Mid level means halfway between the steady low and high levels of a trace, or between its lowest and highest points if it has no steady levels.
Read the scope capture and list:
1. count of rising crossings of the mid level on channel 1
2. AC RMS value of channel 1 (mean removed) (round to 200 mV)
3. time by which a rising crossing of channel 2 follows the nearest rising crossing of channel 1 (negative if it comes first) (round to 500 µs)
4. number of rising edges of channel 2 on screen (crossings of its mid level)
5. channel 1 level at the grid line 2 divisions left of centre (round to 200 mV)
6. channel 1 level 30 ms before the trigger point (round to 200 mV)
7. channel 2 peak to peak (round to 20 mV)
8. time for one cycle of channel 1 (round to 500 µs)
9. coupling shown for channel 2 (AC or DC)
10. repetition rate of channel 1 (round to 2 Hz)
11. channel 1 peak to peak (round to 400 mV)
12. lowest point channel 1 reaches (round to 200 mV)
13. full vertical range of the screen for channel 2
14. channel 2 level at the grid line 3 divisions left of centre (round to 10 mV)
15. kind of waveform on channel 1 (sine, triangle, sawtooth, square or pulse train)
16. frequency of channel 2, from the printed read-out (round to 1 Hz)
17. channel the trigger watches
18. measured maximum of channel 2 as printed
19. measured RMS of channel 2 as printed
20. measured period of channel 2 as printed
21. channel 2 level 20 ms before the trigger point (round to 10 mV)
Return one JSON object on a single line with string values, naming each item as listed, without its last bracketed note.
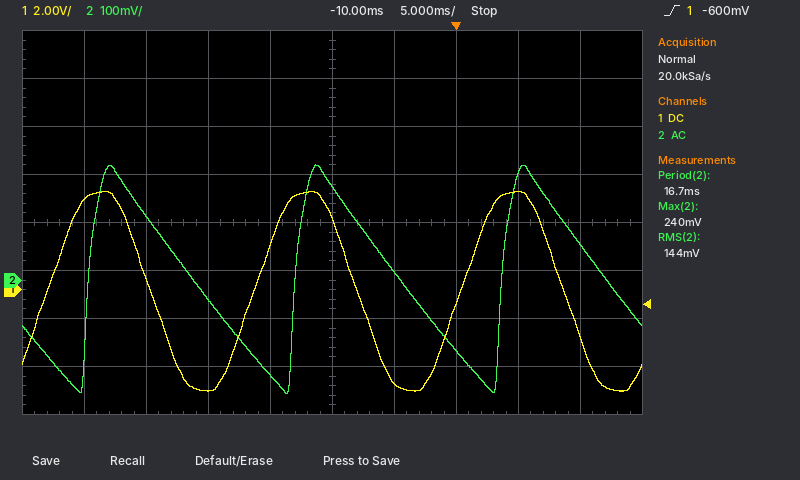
{"count of rising crossings of the mid level on channel 1": "3", "AC RMS value of channel 1 (mean removed)": "3.0 V", "time by which a rising crossing of channel 2 follows the nearest rising crossing of channel 1 (negative if it comes first)": "+3.5 ms", "number of rising edges of channel 2 on screen": "3", "channel 1 level at the grid line 2 divisions left of centre": "-4.2 V", "channel 1 level 30 ms before the trigger point": "3.8 V", "channel 2 peak to peak": "480 mV", "time for one cycle of channel 1": "16.5 ms", "coupling shown for channel 2": "AC", "repetition rate of channel 1": "60 Hz", "channel 1 peak to peak": "8.4 V", "lowest point channel 1 reaches": "-4.2 V", "full vertical range of the screen for channel 2": "800 mV", "channel 2 level at the grid line 3 divisions left of centre": "130 mV", "kind of waveform on channel 1": "sine", "frequency of channel 2, from the printed read-out": "60 Hz", "channel the trigger watches": "channel 1", "measured maximum of channel 2 as printed": "240 mV", "measured RMS of channel 2 as printed": "144 mV", "measured period of channel 2 as printed": "16.7 ms", "channel 2 level 20 ms before the trigger point": "-40 mV"}
